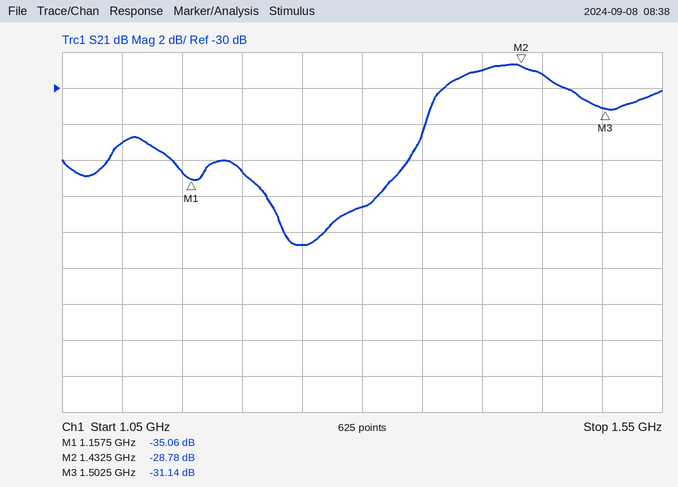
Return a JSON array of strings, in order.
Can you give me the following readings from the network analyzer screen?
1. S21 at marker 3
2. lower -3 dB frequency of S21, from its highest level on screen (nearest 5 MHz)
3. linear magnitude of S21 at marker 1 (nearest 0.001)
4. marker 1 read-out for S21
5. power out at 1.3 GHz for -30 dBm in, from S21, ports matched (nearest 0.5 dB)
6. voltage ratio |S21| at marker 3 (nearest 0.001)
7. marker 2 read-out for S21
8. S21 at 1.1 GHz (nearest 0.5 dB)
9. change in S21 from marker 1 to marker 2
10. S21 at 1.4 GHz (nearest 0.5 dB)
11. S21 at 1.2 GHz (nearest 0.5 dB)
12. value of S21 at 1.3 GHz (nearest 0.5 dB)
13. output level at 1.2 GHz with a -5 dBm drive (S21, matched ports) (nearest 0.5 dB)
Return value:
["-31.14 dB", "1.355 GHz", "0.018", "-35.06 dB", "-66.5 dBm", "0.028", "-28.78 dB", "-33.0 dB", "6.28 dB", "-29.0 dB", "-34.5 dB", "-36.5 dB", "-39.5 dBm"]
